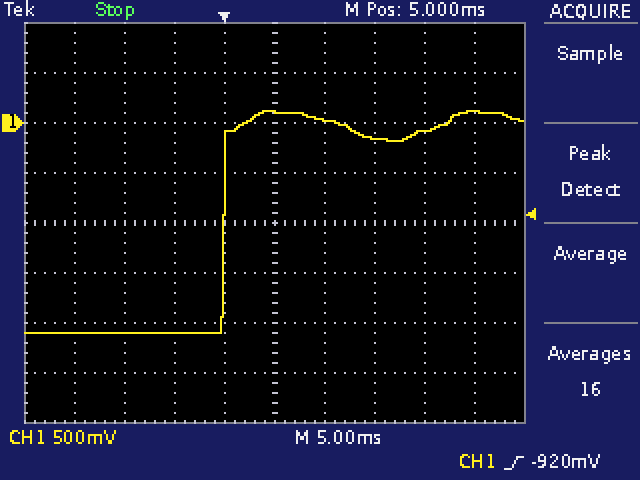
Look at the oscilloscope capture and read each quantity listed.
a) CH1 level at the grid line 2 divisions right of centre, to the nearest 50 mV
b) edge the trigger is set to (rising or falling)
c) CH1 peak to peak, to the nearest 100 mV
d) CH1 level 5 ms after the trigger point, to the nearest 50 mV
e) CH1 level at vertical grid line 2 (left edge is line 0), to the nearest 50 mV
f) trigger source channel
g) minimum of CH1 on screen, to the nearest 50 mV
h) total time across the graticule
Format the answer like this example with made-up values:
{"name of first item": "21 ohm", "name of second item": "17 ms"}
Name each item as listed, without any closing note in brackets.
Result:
{"CH1 level at the grid line 2 divisions right of centre, to the nearest 50 mV": "-150 mV", "edge the trigger is set to": "rising", "CH1 peak to peak, to the nearest 100 mV": "2.20 V", "CH1 level 5 ms after the trigger point, to the nearest 50 mV": "100 mV", "CH1 level at vertical grid line 2 (left edge is line 0), to the nearest 50 mV": "-2.10 V", "trigger source channel": "CH1", "minimum of CH1 on screen, to the nearest 50 mV": "-2.10 V", "total time across the graticule": "50 ms"}
